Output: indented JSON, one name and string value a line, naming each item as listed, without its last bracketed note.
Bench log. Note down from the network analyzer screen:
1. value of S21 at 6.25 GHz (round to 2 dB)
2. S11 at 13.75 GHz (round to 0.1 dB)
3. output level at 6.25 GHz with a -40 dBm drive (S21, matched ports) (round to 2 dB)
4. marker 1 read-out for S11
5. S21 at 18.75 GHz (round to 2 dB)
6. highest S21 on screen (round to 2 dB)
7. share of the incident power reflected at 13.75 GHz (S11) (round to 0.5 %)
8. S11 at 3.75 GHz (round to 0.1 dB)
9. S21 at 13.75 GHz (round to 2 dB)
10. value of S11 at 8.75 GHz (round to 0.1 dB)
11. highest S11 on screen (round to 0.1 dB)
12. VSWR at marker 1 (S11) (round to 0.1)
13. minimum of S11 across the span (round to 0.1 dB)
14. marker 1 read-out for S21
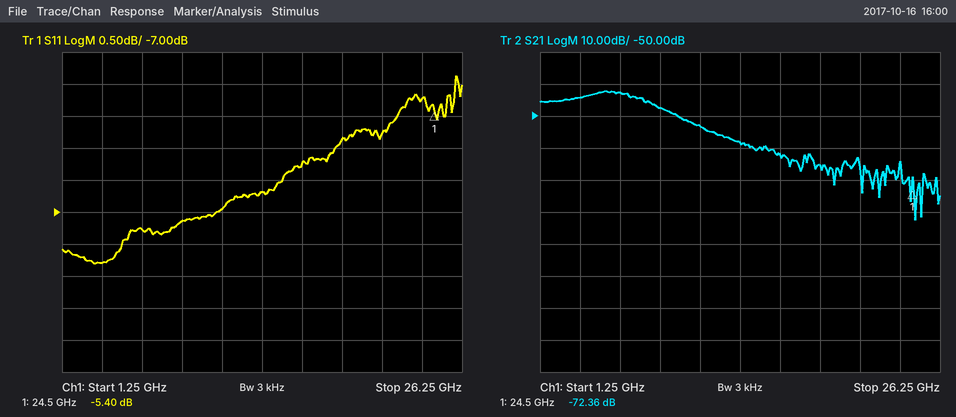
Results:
{
  "value of S21 at 6.25 GHz": "-42 dB",
  "S11 at 13.75 GHz": "-6.7 dB",
  "output level at 6.25 GHz with a -40 dBm drive (S21, matched ports)": "-82 dBm",
  "marker 1 read-out for S11": "-5.40 dB",
  "S21 at 18.75 GHz": "-66 dB",
  "highest S21 on screen": "-42 dB",
  "share of the incident power reflected at 13.75 GHz (S11)": "21.5 %",
  "S11 at 3.75 GHz": "-7.8 dB",
  "S21 at 13.75 GHz": "-58 dB",
  "value of S11 at 8.75 GHz": "-7.1 dB",
  "highest S11 on screen": "-4.9 dB",
  "VSWR at marker 1 (S11)": "3.3",
  "minimum of S11 across the span": "-7.8 dB",
  "marker 1 read-out for S21": "-72.36 dB"
}
